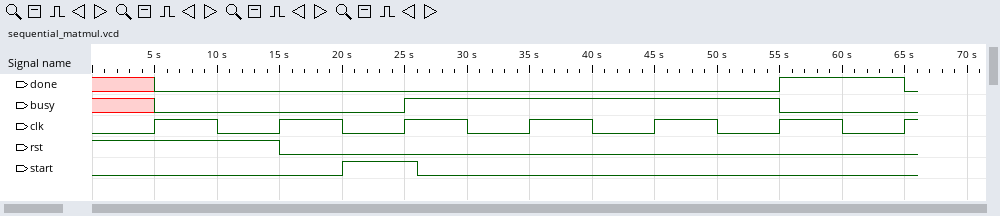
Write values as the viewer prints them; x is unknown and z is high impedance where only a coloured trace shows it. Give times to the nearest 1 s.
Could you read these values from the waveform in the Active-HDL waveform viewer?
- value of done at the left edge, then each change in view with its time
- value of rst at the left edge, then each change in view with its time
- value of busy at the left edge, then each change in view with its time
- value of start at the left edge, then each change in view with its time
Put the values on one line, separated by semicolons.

x, 0 at 5 s, 1 at 55 s, 0 at 65 s; 1, 0 at 15 s; x, 0 at 5 s, 1 at 25 s, 0 at 55 s; 0, 1 at 20 s, 0 at 26 s
